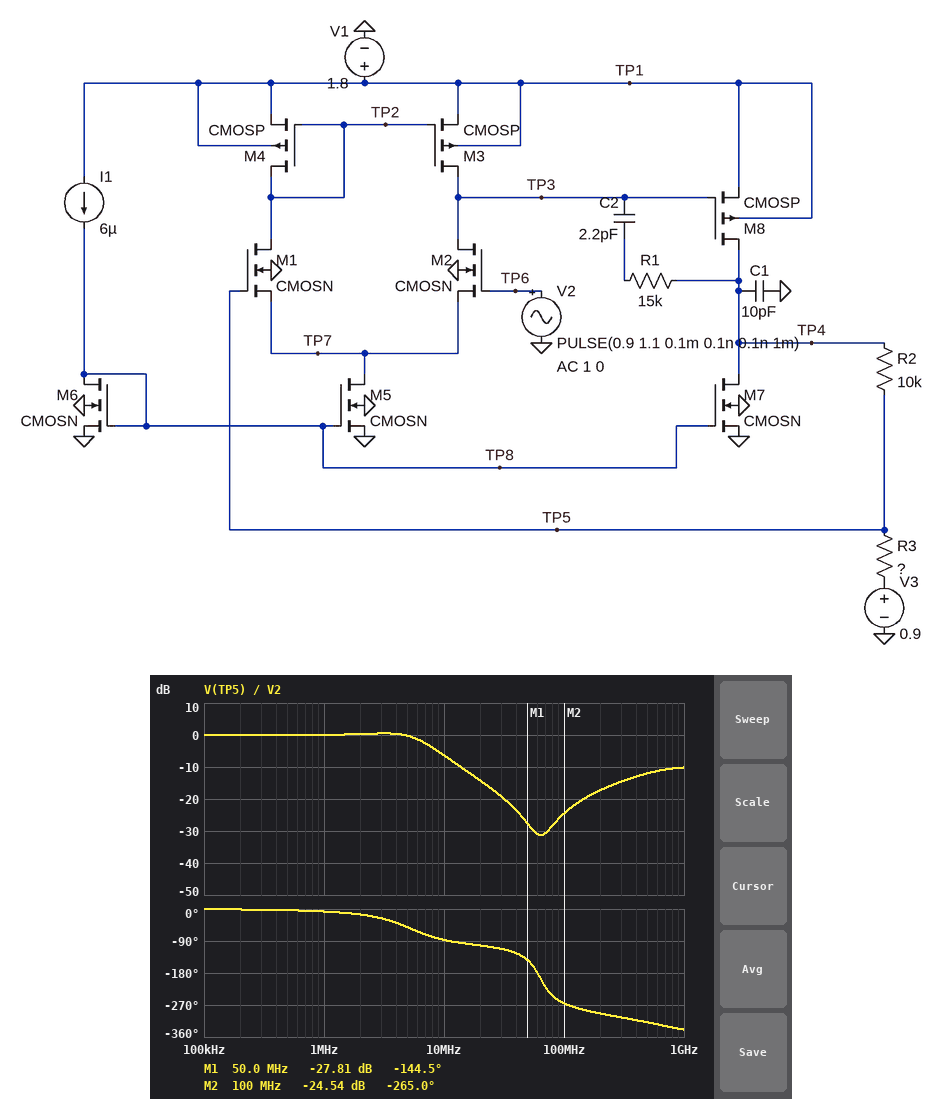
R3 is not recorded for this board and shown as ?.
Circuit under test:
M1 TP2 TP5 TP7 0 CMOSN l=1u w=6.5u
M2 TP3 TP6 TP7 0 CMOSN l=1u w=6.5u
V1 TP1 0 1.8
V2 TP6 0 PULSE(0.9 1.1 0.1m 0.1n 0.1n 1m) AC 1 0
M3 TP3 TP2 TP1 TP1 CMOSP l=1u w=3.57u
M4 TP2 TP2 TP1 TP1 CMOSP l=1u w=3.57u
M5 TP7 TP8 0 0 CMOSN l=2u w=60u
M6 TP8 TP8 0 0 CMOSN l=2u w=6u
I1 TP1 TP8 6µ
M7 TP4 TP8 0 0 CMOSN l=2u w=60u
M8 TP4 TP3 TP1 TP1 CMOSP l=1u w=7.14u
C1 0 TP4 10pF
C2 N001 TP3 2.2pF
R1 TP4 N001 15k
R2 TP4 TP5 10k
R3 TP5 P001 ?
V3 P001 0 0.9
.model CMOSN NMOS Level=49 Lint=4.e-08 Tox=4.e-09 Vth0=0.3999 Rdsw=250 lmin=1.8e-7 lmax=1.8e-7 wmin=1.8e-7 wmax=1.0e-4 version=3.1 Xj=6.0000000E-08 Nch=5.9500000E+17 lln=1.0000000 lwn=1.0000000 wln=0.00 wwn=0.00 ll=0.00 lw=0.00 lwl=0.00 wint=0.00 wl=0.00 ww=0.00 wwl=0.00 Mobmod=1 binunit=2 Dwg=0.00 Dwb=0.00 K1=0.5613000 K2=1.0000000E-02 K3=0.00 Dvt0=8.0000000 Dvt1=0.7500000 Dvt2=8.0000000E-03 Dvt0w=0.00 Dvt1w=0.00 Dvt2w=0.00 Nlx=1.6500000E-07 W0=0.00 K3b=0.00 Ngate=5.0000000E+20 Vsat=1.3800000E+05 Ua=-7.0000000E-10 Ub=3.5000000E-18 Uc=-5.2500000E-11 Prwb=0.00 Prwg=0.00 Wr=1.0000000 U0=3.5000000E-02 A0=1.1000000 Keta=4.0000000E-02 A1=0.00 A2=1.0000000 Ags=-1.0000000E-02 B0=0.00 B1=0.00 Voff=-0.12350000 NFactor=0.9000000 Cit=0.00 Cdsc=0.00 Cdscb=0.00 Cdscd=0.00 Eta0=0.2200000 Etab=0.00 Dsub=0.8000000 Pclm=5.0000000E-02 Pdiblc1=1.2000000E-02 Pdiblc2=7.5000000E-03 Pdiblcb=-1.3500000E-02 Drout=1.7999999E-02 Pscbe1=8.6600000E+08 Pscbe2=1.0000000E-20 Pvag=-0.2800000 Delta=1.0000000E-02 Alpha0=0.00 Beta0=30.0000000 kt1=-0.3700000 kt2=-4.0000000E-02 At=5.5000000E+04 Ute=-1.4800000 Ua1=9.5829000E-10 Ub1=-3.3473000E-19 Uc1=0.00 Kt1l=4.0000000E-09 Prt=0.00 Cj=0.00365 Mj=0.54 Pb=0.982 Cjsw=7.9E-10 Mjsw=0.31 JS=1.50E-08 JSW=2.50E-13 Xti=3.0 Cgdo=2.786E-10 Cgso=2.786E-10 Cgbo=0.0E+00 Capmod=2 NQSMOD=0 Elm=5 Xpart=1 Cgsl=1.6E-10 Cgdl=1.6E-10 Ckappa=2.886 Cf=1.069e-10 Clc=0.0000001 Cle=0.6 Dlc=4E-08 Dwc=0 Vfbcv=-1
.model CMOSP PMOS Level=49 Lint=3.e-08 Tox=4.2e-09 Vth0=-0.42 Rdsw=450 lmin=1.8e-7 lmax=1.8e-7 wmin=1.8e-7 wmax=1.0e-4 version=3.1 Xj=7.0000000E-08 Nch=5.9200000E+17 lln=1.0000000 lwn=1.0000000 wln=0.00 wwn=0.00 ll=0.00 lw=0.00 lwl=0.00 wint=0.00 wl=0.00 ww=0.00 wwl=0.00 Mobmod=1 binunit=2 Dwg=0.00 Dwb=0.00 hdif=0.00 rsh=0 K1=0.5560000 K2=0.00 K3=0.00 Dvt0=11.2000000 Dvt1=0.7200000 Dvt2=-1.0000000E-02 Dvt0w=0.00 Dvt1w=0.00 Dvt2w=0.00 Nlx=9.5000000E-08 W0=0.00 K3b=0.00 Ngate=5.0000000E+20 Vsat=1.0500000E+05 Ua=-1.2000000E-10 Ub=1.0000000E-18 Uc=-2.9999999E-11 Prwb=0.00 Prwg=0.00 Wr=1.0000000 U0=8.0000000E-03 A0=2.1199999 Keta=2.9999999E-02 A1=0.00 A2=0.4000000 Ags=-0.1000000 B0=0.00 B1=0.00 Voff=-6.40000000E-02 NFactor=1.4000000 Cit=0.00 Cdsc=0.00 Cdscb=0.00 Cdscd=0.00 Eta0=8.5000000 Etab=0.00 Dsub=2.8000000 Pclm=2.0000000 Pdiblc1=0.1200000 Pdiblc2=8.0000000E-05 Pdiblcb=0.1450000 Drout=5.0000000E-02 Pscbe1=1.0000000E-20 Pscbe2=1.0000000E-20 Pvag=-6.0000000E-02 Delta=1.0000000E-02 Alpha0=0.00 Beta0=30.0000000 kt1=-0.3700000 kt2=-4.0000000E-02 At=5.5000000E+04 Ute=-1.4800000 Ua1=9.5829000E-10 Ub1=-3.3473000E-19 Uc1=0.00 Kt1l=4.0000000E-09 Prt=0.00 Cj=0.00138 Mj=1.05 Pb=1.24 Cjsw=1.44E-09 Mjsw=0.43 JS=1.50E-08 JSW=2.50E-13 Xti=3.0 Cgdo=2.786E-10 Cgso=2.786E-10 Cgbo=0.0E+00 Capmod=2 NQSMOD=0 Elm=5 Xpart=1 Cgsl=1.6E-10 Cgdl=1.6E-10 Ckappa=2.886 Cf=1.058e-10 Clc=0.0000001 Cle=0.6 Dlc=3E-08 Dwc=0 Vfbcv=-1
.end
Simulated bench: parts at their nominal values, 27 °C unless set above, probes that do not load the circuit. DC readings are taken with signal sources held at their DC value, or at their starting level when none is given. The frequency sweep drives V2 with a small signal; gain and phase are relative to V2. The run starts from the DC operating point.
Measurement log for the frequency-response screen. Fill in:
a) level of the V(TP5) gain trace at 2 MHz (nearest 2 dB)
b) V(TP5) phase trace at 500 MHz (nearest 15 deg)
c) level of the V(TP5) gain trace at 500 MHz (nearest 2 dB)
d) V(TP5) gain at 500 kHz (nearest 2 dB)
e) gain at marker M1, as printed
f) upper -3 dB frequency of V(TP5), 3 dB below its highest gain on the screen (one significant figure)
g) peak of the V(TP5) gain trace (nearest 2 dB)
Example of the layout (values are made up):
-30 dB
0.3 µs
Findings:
0 dB
-315 deg
-12 dB
0 dB
-27.81 dB
7 MHz
0 dB
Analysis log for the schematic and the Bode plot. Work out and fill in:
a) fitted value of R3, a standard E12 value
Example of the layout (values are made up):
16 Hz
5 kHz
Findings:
18 kΩ
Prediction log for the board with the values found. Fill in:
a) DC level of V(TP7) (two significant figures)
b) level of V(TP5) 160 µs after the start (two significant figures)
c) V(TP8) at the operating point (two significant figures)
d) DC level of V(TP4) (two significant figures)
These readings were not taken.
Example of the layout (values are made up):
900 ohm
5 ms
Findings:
220 mV
1.1 V
520 mV
900 mV
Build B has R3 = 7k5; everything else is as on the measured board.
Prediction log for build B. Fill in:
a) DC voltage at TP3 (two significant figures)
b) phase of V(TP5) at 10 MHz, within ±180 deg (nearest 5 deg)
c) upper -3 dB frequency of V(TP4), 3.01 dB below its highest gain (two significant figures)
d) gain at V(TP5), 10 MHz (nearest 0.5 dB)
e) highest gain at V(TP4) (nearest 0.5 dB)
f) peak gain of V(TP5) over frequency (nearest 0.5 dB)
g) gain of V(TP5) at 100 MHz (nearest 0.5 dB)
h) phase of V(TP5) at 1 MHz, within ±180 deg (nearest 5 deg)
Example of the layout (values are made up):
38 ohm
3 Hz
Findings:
730 mV
-95 deg
5.2 MHz
-10.0 dB
7.5 dB
0 dB
-28.0 dB
-10 deg
